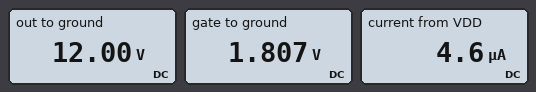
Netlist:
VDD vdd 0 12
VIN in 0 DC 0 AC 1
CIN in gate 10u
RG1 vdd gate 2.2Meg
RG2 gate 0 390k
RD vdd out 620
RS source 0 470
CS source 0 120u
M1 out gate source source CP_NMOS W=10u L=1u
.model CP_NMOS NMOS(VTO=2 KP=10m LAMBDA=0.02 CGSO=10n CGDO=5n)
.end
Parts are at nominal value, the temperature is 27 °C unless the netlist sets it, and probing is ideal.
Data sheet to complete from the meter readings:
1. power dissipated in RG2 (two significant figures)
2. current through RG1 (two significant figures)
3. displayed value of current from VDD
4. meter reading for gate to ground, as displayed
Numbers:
8.4 µW
4.6 µA
4.6 µA
1.807 V
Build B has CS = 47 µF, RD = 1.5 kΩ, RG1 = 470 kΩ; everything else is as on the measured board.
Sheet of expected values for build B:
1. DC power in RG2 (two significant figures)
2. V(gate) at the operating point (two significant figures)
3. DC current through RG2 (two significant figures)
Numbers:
76 µW
5.4 V
14 µA
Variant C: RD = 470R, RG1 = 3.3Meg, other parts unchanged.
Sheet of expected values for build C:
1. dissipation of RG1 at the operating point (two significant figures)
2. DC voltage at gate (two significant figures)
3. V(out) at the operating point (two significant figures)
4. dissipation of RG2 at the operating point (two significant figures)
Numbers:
35 µW
1.3 V
12 V
4.1 µW
